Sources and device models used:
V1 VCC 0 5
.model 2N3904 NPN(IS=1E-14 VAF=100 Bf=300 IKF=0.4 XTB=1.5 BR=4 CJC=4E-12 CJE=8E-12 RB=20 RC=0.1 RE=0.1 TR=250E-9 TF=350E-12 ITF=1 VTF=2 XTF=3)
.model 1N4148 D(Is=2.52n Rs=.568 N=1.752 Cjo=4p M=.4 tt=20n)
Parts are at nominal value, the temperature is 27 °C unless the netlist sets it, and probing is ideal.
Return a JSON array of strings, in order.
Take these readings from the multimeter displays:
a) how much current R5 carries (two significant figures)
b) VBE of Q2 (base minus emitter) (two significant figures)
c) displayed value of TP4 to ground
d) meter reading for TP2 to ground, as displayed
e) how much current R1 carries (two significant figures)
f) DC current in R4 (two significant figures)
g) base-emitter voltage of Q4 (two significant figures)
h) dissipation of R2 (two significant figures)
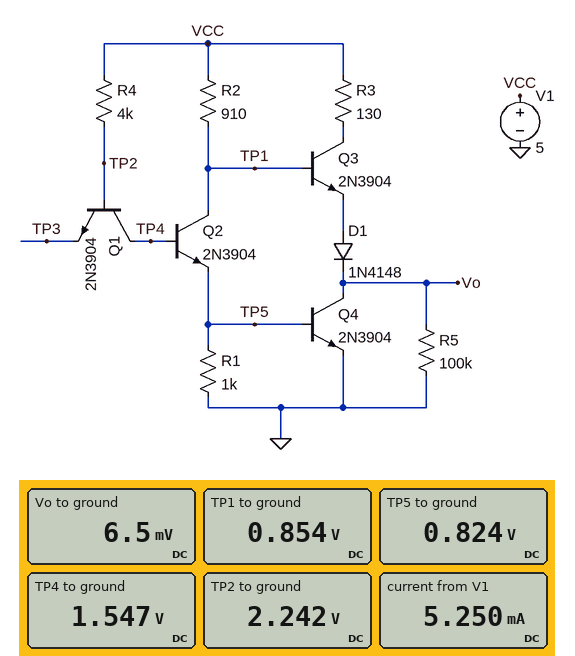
["65 nA", "720 mV", "1.547 V", "2.242 V", "820 µA", "690 µA", "820 mV", "19 mW"]
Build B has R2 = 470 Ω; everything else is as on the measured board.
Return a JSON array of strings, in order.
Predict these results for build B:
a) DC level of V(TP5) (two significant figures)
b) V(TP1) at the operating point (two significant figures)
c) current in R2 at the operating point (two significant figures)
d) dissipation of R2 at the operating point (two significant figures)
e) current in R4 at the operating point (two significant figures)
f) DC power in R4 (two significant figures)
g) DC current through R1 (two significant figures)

["920 mV", "960 mV", "8.6 mA", "35 mW", "660 µA", "1.8 mW", "920 µA"]
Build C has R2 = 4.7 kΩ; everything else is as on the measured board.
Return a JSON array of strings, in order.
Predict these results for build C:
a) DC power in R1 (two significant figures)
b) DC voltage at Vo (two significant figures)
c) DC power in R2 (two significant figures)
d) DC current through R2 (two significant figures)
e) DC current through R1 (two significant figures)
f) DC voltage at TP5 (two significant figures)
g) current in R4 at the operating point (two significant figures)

["510 µW", "6.0 mV", "3.9 mW", "910 µA", "710 µA", "710 mV", "720 µA"]
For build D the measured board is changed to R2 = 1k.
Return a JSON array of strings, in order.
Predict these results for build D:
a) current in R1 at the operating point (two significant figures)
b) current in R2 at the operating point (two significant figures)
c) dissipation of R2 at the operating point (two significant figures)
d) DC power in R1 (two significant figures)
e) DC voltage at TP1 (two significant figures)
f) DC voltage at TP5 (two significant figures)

["810 µA", "4.2 mA", "17 mW", "660 µW", "840 mV", "810 mV"]
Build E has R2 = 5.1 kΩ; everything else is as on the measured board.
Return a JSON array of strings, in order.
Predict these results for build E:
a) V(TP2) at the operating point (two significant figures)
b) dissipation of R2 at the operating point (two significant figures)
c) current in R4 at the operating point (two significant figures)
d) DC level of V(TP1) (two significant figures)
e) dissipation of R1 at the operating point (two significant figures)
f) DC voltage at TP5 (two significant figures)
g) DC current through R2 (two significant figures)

["2.1 V", "3.6 mW", "720 µA", "720 mV", "500 µW", "710 mV", "840 µA"]
